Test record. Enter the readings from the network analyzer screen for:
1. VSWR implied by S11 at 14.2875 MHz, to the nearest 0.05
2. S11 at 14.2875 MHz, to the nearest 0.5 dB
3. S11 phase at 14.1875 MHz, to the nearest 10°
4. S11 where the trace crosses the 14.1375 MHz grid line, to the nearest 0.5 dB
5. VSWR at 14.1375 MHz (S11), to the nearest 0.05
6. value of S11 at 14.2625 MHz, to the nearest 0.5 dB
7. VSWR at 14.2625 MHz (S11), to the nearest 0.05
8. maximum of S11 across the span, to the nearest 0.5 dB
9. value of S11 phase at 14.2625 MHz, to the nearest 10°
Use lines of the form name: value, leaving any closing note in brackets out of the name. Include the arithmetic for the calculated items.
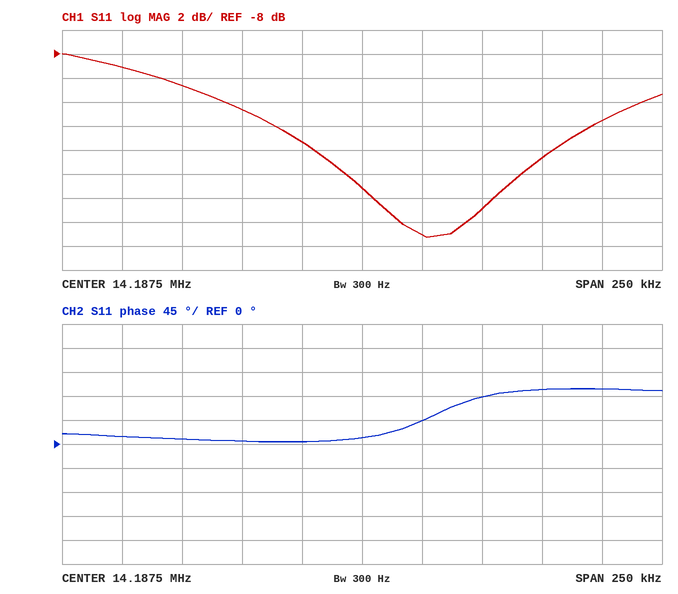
VSWR implied by S11 at 14.2875 MHz, to the nearest 0.05: |Γ| = 10^(-13.5/20) = 0.2113; VSWR = (1 + 0.2113)/(1 − 0.2113) ≈ 1.54, so 1.55 to the nearest 0.05
S11 at 14.2875 MHz, to the nearest 0.5 dB: -13.5 dB
S11 phase at 14.1875 MHz, to the nearest 10°: 10°
S11 where the trace crosses the 14.1375 MHz grid line, to the nearest 0.5 dB: -12.5 dB
VSWR at 14.1375 MHz (S11), to the nearest 0.05: |Γ| = 10^(-12.5/20) = 0.2371; VSWR = (1 + 0.2371)/(1 − 0.2371) ≈ 1.62, so 1.60 to the nearest 0.05
value of S11 at 14.2625 MHz, to the nearest 0.5 dB: -16.5 dB
VSWR at 14.2625 MHz (S11), to the nearest 0.05: |Γ| = 10^(-16.5/20) = 0.1496; VSWR = (1 + 0.1496)/(1 − 0.1496) ≈ 1.35
maximum of S11 across the span, to the nearest 0.5 dB: -8.0 dB
value of S11 phase at 14.2625 MHz, to the nearest 10°: 100°
